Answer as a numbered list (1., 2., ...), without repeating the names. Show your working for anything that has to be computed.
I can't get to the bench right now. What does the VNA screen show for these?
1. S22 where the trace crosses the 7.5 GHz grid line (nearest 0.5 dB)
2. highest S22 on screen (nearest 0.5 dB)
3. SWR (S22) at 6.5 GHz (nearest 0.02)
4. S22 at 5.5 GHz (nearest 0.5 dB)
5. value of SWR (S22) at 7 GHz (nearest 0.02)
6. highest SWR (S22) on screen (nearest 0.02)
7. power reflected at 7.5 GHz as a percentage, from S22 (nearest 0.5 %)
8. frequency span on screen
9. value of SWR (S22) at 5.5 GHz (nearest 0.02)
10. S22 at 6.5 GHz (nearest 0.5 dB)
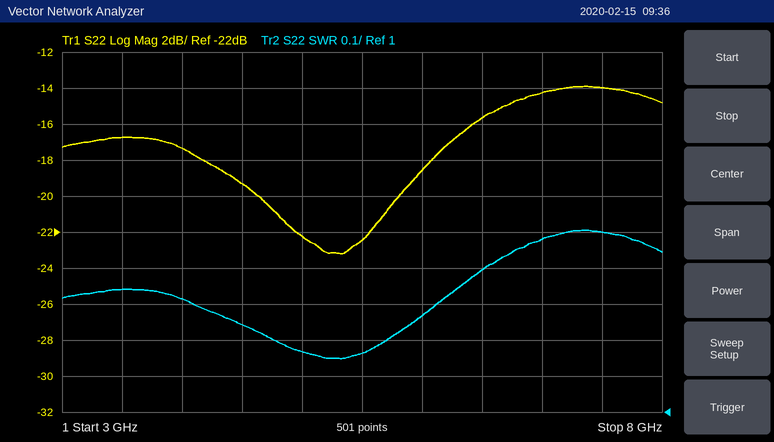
1. -14.0 dB
2. -14.0 dB
3. 1.40
4. -22.5 dB
5. 1.48
6. 1.50
7. 10^(-14/10) ≈ 4.0 %
8. 5 GHz
9. 1.16
10. -15.5 dB
